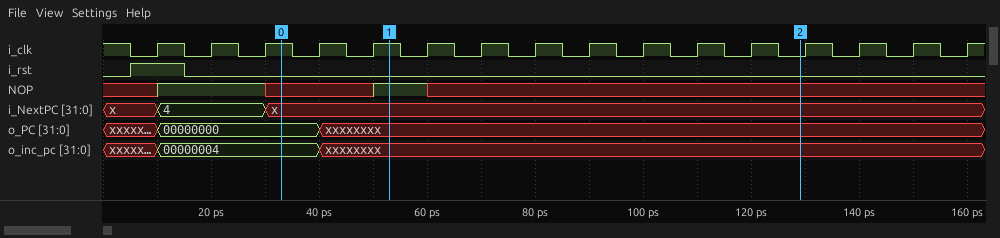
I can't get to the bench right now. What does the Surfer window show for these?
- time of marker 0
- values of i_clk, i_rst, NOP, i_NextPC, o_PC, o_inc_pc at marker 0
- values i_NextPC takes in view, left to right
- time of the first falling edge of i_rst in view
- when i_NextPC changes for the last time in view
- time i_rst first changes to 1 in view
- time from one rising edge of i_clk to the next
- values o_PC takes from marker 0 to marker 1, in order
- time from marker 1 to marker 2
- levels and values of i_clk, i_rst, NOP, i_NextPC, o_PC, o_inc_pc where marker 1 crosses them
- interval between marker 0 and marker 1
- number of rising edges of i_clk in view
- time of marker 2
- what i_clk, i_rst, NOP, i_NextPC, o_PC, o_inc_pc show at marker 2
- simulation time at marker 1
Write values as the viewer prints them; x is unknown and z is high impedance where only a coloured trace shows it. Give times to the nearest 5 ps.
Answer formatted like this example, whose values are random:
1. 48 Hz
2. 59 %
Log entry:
1. 35 ps
2. i_clk=1, i_rst=0, NOP=x, i_NextPC=x, o_PC=00000000, o_inc_pc=00000004
3. x, 4, x
4. 15 ps
5. 30 ps
6. 5 ps
7. 10 ps
8. 00000000, xxxxxxxx
9. 75 ps
10. i_clk=1, i_rst=0, NOP=1, i_NextPC=x, o_PC=xxxxxxxx, o_inc_pc=xxxxxxxx
11. 20 ps
12. 16
13. 130 ps
14. i_clk=0, i_rst=0, NOP=x, i_NextPC=x, o_PC=xxxxxxxx, o_inc_pc=xxxxxxxx
15. 55 ps
